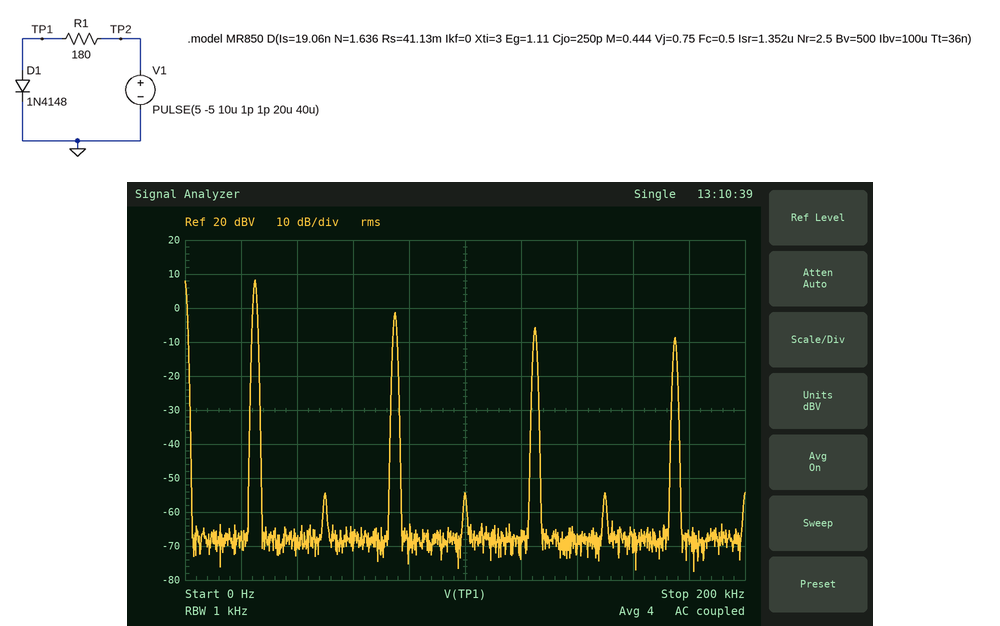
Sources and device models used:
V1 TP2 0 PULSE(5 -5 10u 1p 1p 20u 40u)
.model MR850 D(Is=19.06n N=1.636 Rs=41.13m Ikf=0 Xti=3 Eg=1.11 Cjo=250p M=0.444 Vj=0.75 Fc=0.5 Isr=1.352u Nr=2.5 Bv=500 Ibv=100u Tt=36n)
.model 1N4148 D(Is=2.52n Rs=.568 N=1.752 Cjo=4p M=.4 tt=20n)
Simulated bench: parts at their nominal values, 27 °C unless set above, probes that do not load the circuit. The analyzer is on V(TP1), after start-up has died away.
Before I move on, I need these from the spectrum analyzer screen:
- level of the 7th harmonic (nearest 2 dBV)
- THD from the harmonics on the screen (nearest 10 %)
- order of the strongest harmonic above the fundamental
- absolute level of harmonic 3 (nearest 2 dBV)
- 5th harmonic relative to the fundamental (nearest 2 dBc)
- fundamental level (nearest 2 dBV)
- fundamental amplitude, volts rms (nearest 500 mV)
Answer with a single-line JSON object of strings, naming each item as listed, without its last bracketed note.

{"level of the 7th harmonic": "-8 dBV", "THD from the harmonics on the screen": "40 %", "order of the strongest harmonic above the fundamental": "3", "absolute level of harmonic 3": "-2 dBV", "5th harmonic relative to the fundamental": "-14 dBc", "fundamental level": "8 dBV", "fundamental amplitude, volts rms": "2.5 V"}
